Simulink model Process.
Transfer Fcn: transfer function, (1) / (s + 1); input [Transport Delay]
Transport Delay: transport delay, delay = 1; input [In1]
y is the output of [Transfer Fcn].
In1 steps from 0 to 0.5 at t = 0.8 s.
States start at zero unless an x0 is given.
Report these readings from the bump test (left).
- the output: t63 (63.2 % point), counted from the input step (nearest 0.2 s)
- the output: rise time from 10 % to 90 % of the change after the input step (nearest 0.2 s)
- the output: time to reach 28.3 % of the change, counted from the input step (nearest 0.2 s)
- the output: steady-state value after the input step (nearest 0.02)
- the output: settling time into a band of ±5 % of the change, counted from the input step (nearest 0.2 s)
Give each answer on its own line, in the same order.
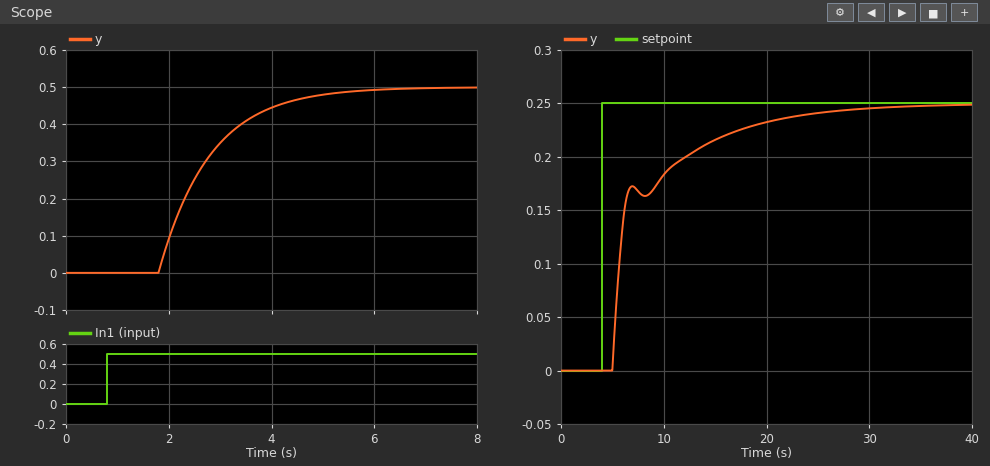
2.0 s
2.2 s
1.4 s
0.50
4.0 s
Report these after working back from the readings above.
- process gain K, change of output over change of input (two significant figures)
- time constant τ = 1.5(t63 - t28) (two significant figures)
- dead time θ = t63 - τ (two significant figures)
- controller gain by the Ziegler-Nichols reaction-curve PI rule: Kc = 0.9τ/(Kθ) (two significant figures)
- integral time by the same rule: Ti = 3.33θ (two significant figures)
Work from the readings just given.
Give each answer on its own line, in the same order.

1.0
0.90 s
1.1 s
0.74
3.7 s
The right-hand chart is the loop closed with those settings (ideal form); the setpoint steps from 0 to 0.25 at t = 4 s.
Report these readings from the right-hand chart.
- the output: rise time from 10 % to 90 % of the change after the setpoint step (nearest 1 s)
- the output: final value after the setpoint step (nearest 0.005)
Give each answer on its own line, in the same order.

12 s
0.250
